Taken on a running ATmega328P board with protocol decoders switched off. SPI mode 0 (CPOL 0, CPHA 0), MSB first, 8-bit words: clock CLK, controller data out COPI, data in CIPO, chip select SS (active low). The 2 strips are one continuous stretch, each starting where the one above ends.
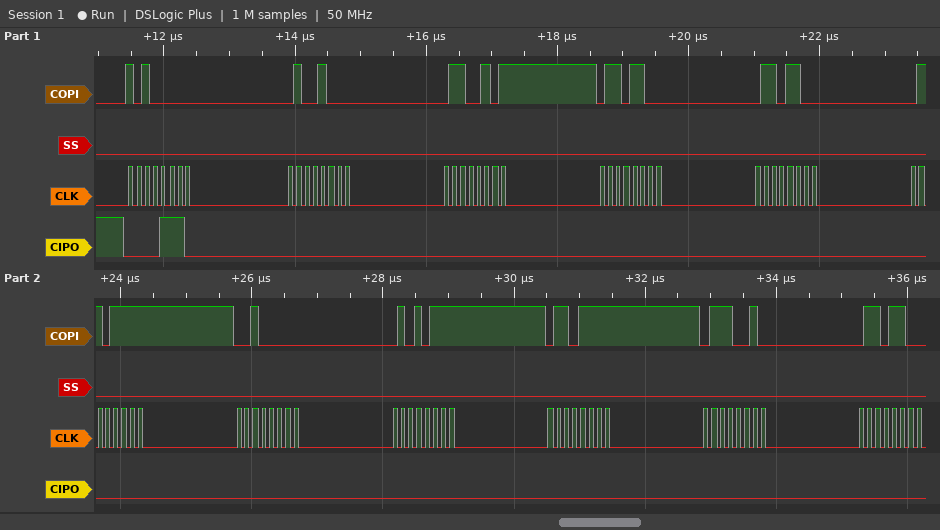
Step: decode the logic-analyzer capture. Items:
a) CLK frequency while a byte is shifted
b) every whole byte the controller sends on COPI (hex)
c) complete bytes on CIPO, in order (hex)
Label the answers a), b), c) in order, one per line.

a) 8 MHz
b) 0xA0 0x48 0x65 0x6C 0x6C 0x6F 0x20 0x57 0x6F 0x72 0x6C
c) 0x0E 0x00 0x00 0x00 0x00 0x00 0x00 0x00 0x00 0x00 0x00
